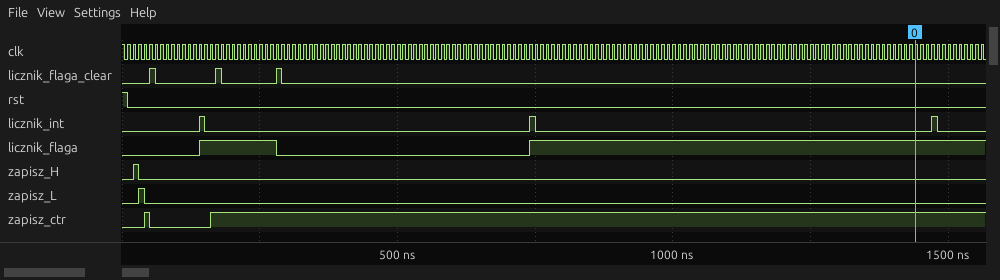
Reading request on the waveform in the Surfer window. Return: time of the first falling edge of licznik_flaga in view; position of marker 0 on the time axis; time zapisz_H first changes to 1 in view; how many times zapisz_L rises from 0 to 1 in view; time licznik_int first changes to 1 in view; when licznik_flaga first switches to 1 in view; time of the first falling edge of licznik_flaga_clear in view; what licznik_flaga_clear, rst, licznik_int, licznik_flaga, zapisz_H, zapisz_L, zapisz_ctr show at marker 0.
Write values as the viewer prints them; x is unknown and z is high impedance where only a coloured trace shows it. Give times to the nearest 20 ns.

280 ns
1440 ns
20 ns
1
140 ns
140 ns
60 ns
licznik_flaga_clear=0, rst=0, licznik_int=0, licznik_flaga=1, zapisz_H=0, zapisz_L=0, zapisz_ctr=1
